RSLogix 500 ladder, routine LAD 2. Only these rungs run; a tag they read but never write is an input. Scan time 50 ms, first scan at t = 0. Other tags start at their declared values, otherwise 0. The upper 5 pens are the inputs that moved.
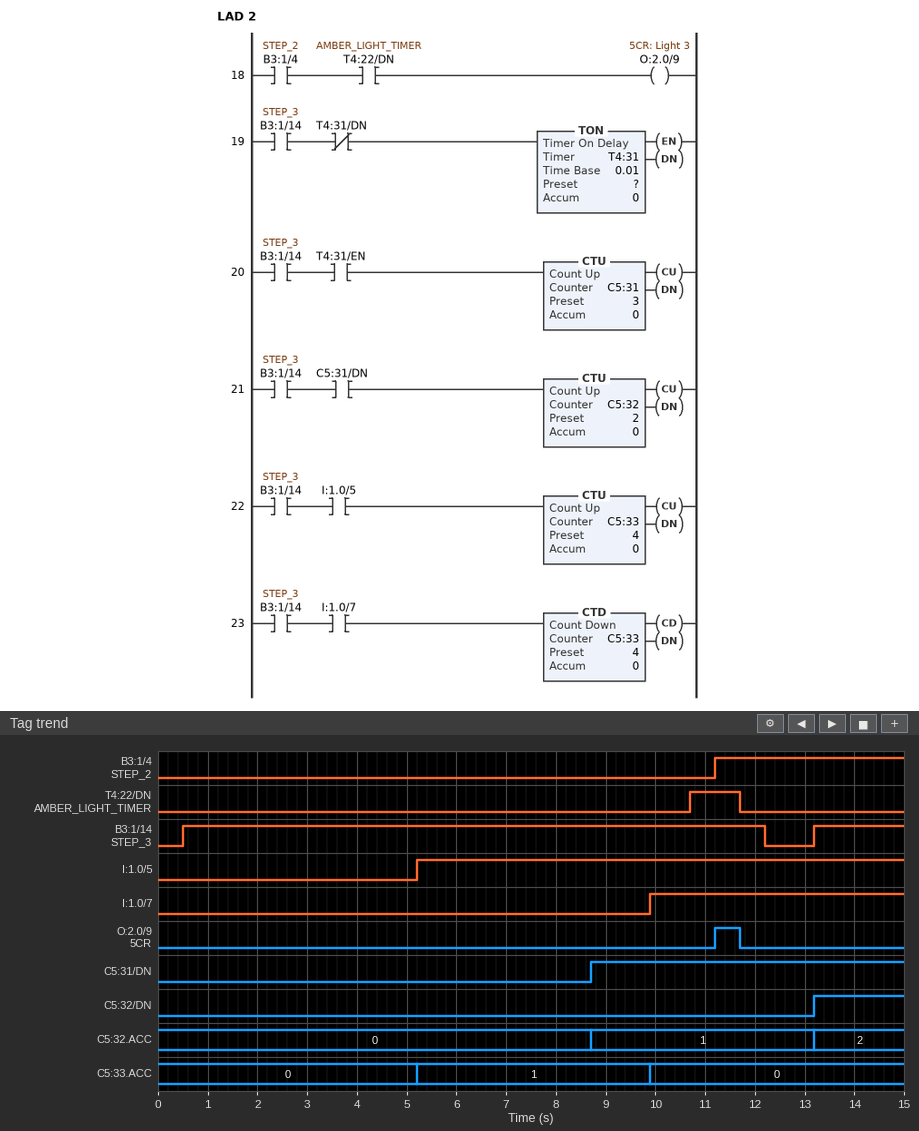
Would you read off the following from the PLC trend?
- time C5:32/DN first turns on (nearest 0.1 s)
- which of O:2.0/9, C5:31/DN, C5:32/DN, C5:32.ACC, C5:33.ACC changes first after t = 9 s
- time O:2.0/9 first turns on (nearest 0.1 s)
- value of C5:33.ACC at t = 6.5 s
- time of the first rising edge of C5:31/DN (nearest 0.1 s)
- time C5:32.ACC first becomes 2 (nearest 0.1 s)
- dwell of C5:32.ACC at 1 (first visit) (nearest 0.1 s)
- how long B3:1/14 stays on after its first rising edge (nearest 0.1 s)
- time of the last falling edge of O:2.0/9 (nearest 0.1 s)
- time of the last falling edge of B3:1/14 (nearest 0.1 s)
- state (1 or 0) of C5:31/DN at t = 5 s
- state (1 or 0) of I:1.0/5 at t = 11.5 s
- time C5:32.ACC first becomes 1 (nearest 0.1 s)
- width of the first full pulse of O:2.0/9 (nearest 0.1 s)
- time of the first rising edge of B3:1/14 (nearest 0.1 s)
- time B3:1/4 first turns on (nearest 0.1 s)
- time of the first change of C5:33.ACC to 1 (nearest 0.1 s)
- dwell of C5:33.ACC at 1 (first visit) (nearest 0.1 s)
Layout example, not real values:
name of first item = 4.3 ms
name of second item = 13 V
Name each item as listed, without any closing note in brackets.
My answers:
time C5:32/DN first turns on = 13.2 s
which of O:2.0/9, C5:31/DN, C5:32/DN, C5:32.ACC, C5:33.ACC changes first after t = 9 s = C5:33.ACC
time O:2.0/9 first turns on = 11.2 s
value of C5:33.ACC at t = 6.5 s = 1
time of the first rising edge of C5:31/DN = 8.7 s
time C5:32.ACC first becomes 2 = 13.2 s
dwell of C5:32.ACC at 1 (first visit) = 4.5 s
how long B3:1/14 stays on after its first rising edge = 11.7 s
time of the last falling edge of O:2.0/9 = 11.7 s
time of the last falling edge of B3:1/14 = 12.2 s
state (1 or 0) of C5:31/DN at t = 5 s = 0
state (1 or 0) of I:1.0/5 at t = 11.5 s = 1
time C5:32.ACC first becomes 1 = 8.7 s
width of the first full pulse of O:2.0/9 = 0.5 s
time of the first rising edge of B3:1/14 = 0.5 s
time B3:1/4 first turns on = 11.2 s
time of the first change of C5:33.ACC to 1 = 5.2 s
dwell of C5:33.ACC at 1 (first visit) = 4.7 s
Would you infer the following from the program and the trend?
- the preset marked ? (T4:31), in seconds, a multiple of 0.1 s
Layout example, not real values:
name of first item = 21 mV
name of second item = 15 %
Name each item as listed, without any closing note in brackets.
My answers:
the preset marked ? (T4:31), in seconds, a multiple of 0.1 s = 4.0 s
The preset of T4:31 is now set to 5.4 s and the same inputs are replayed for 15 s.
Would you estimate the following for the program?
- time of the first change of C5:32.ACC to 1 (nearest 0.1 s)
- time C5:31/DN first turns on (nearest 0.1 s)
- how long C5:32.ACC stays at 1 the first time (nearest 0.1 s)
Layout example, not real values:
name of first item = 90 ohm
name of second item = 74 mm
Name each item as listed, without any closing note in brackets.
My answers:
time of the first change of C5:32.ACC to 1 = 11.5 s
time C5:31/DN first turns on = 11.5 s
how long C5:32.ACC stays at 1 the first time = 1.7 s
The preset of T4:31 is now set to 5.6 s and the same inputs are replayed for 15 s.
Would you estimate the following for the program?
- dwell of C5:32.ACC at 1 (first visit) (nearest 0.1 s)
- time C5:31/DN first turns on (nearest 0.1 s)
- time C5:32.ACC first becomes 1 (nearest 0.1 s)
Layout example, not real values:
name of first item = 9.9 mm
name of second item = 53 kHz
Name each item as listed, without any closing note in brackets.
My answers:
dwell of C5:32.ACC at 1 (first visit) = 1.3 s
time C5:31/DN first turns on = 11.9 s
time C5:32.ACC first becomes 1 = 11.9 s
